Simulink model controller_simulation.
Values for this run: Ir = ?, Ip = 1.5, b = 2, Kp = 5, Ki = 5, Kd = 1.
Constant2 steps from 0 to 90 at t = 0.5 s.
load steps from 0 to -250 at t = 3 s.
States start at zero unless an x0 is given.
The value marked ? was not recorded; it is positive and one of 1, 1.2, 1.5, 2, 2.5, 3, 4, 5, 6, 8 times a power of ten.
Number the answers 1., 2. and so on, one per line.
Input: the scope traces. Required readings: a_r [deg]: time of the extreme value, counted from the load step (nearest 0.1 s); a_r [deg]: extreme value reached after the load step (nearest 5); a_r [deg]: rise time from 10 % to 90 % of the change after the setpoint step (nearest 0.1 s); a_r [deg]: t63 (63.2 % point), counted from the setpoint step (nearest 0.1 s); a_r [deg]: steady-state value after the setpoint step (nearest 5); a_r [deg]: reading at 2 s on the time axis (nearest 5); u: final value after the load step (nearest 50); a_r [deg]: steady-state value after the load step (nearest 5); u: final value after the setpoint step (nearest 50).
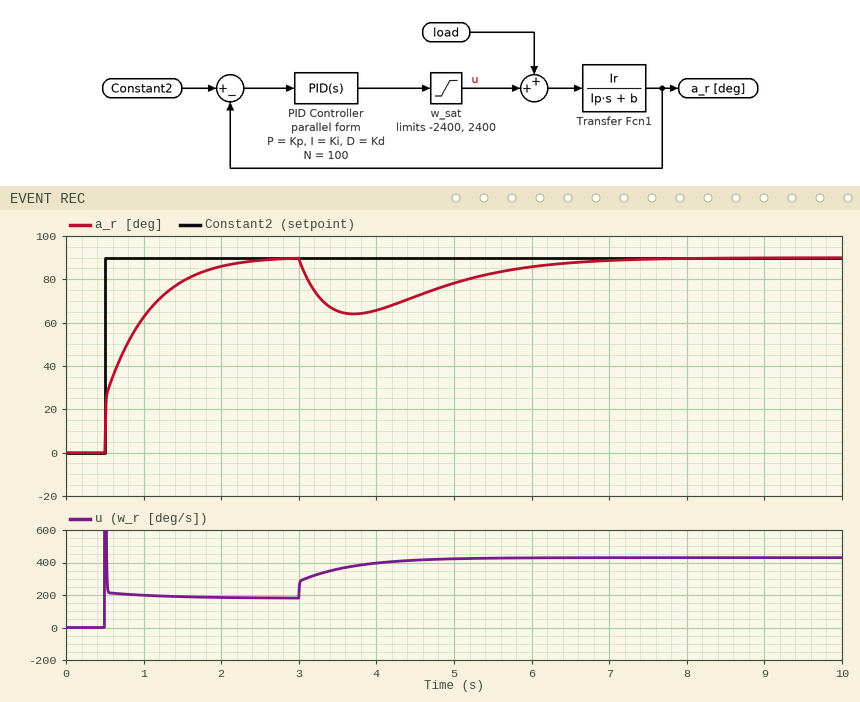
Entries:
1. 0.7 s
2. 65
3. 1.1 s
4. 0.4 s
5. 90
6. 85
7. 450
8. 90
9. 200
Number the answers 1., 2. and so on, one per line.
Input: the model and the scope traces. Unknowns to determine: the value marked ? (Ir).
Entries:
1. 1
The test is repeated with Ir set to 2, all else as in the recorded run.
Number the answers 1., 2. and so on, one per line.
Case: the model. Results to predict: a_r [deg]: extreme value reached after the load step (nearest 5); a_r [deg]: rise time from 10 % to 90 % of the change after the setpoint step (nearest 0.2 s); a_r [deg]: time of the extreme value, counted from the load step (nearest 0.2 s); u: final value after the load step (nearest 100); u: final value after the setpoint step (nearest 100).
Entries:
1. 60
2. 0.6 s
3. 0.6 s
4. 300
5. 100
